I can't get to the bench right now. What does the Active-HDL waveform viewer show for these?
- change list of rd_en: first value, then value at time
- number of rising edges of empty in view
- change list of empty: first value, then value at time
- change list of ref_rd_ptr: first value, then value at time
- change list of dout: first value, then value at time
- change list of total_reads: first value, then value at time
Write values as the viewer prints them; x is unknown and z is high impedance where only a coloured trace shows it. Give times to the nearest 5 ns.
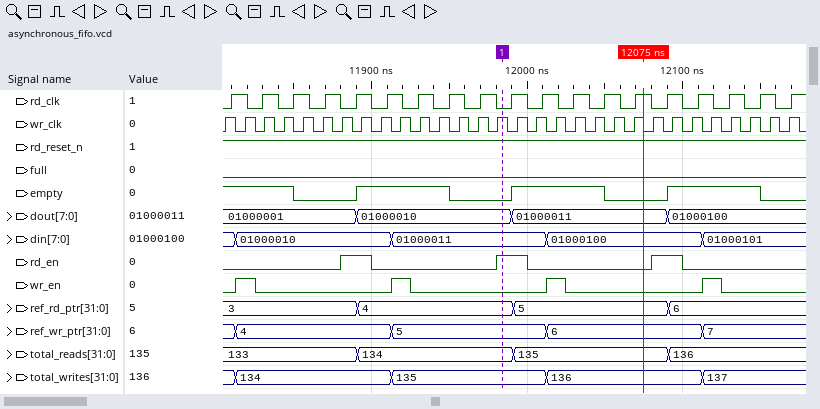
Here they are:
0, 1 at 11880 ns, 0 at 11900 ns, 1 at 11980 ns, 0 at 12000 ns, 1 at 12080 ns, 0 at 12100 ns
3
1, 0 at 11850 ns, 1 at 11890 ns, 0 at 11950 ns, 1 at 11990 ns, 0 at 12050 ns, 1 at 12090 ns, 0 at 12150 ns
3, 4 at 11890 ns, 5 at 11990 ns, 6 at 12090 ns
01000001, 01000010 at 11890 ns, 01000011 at 11990 ns, 01000100 at 12090 ns
133, 134 at 11890 ns, 135 at 11990 ns, 136 at 12090 ns
